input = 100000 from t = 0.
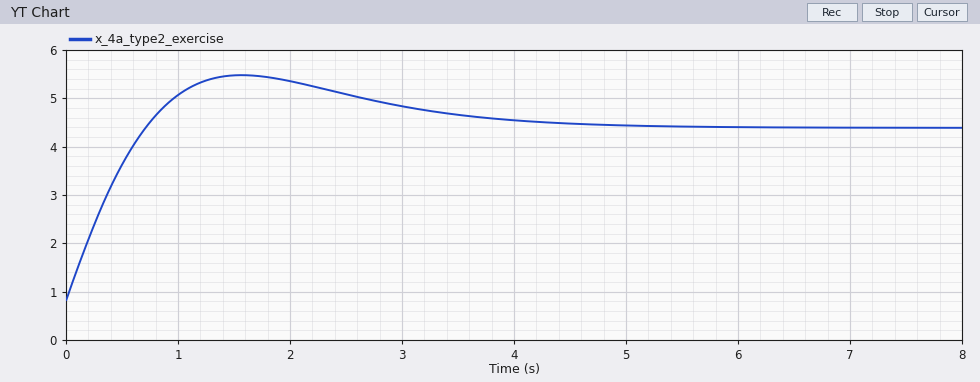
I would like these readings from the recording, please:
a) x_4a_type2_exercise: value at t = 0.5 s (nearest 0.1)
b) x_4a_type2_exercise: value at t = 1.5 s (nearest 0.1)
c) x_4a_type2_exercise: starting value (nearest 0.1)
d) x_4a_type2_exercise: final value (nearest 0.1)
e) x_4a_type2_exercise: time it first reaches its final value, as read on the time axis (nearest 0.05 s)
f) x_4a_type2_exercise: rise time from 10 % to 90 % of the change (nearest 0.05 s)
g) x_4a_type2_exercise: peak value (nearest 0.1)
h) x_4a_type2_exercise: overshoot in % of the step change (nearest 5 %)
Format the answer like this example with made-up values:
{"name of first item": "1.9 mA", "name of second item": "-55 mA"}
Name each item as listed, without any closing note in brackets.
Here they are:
{"x_4a_type2_exercise: value at t = 0.5 s": "3.6", "x_4a_type2_exercise: value at t = 1.5 s": "5.5", "x_4a_type2_exercise: starting value": "0.8", "x_4a_type2_exercise: final value": "4.4", "x_4a_type2_exercise: time it first reaches its final value, as read on the time axis": "0.70 s", "x_4a_type2_exercise: rise time from 10 % to 90 % of the change": "0.55 s", "x_4a_type2_exercise: peak value": "5.5", "x_4a_type2_exercise: overshoot in % of the step change": "30 %"}
